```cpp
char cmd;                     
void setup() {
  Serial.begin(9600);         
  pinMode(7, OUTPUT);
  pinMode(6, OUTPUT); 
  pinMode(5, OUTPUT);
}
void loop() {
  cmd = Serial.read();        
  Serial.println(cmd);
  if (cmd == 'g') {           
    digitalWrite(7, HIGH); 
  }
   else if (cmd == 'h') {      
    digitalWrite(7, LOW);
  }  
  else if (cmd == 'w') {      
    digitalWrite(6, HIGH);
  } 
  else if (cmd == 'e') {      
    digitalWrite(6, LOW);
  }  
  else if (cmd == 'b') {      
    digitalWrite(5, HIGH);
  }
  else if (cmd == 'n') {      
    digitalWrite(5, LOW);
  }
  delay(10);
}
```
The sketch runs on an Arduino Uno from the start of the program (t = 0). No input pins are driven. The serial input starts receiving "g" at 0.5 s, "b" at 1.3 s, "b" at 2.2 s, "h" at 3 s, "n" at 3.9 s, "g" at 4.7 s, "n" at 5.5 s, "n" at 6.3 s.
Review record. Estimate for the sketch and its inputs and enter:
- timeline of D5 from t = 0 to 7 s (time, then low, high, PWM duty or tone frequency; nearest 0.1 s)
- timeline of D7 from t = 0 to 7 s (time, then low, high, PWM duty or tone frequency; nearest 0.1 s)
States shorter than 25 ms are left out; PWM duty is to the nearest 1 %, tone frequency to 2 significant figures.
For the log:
0 s low; 1.3 s high; 3.9 s low
0 s low; 0.5 s high; 3 s low; 4.7 s high
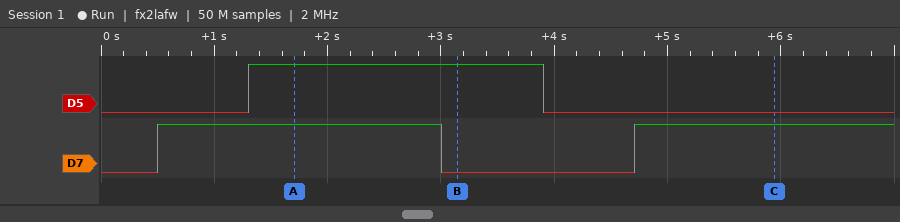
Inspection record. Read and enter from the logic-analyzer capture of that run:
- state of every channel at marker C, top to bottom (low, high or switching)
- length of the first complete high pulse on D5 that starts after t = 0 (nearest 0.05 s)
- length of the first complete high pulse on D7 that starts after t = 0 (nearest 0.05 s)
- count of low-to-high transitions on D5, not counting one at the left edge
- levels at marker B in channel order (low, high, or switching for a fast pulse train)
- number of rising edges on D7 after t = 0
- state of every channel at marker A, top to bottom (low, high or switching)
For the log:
D5 low, D7 high
2.60 s
2.50 s
1
D5 high, D7 low
2
D5 high, D7 high
